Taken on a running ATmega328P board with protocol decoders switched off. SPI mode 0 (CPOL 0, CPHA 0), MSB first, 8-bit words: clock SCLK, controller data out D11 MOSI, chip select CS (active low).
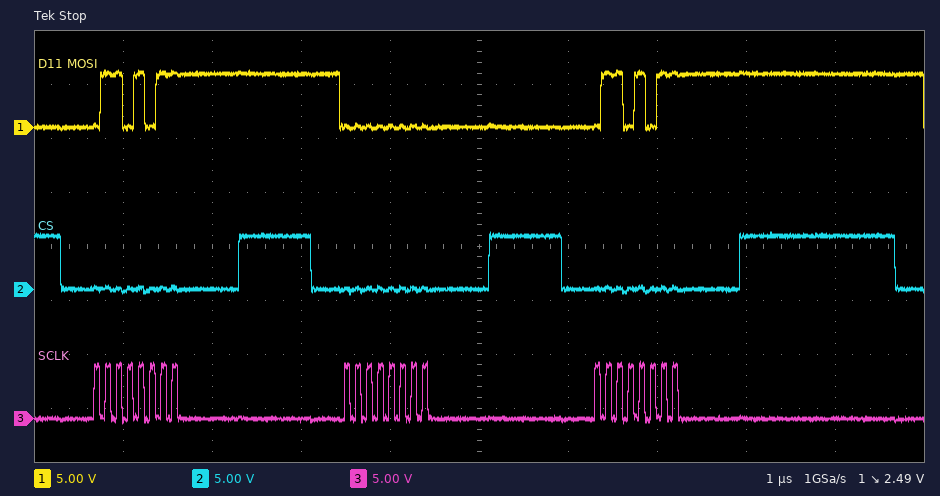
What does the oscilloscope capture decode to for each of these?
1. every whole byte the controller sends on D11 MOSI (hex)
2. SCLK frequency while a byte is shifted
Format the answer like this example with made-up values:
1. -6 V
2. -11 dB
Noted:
1. 0x6B 0x00 0x6B
2. 8 MHz
